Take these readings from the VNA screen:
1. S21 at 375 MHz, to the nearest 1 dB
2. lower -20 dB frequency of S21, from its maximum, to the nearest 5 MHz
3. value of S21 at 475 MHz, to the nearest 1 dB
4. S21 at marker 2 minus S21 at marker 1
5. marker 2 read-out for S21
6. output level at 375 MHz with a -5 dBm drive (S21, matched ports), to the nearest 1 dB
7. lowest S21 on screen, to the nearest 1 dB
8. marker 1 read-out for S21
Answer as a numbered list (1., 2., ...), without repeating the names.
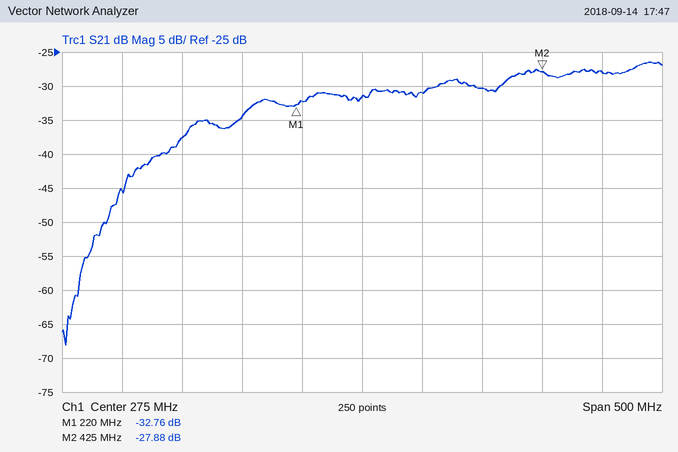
1. -30 dB
2. 70 MHz
3. -28 dB
4. 4.88 dB
5. -27.88 dB
6. -35 dBm
7. -68 dB
8. -32.76 dB
